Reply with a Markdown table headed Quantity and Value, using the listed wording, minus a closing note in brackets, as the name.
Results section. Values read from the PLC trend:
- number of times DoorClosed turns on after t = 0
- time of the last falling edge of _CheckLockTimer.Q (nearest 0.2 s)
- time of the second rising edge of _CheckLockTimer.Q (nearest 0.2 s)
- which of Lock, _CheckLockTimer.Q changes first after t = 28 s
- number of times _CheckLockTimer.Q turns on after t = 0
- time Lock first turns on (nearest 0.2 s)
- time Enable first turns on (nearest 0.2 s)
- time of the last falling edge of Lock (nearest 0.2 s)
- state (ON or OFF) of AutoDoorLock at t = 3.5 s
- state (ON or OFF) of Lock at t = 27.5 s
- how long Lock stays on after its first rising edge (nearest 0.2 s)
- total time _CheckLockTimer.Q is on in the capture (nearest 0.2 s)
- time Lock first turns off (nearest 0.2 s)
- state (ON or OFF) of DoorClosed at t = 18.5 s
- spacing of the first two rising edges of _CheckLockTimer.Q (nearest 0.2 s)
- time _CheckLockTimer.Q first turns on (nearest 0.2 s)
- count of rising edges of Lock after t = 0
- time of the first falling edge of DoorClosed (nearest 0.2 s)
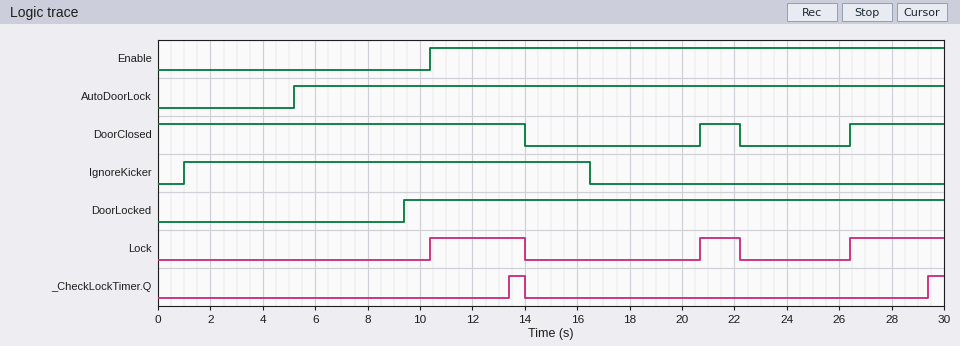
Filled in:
| Quantity | Value |
|---|---|
| number of times DoorClosed turns on after t = 0 | 2 |
| time of the last falling edge of _CheckLockTimer.Q | 14.0 s |
| time of the second rising edge of _CheckLockTimer.Q | 29.4 s |
| which of Lock, _CheckLockTimer.Q changes first after t = 28 s | _CheckLockTimer.Q |
| number of times _CheckLockTimer.Q turns on after t = 0 | 2 |
| time Lock first turns on | 10.4 s |
| time Enable first turns on | 10.4 s |
| time of the last falling edge of Lock | 22.2 s |
| state (ON or OFF) of AutoDoorLock at t = 3.5 s | OFF |
| state (ON or OFF) of Lock at t = 27.5 s | ON |
| how long Lock stays on after its first rising edge | 3.6 s |
| total time _CheckLockTimer.Q is on in the capture | 1.2 s |
| time Lock first turns off | 14.0 s |
| state (ON or OFF) of DoorClosed at t = 18.5 s | OFF |
| spacing of the first two rising edges of _CheckLockTimer.Q | 16.0 s |
| time _CheckLockTimer.Q first turns on | 13.4 s |
| count of rising edges of Lock after t = 0 | 3 |
| time of the first falling edge of DoorClosed | 14.0 s |
